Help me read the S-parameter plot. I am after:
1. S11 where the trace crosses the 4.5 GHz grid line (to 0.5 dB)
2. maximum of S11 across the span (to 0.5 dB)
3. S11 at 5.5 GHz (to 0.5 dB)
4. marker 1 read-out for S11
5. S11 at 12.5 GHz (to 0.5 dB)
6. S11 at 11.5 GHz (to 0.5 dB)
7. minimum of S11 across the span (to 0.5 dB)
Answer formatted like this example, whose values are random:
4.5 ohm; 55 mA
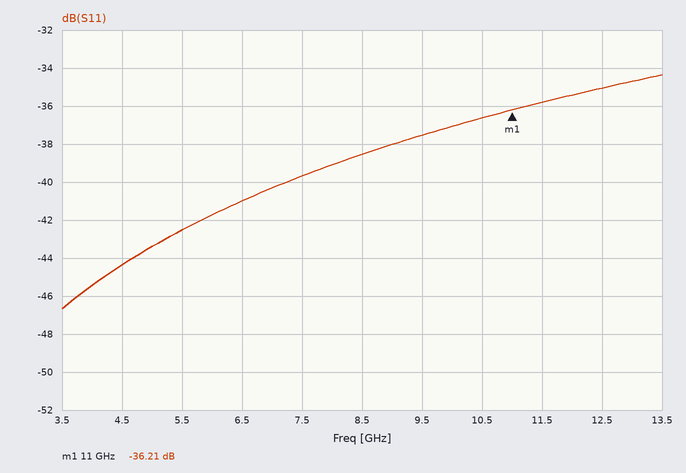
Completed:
-44.5 dB; -34.5 dB; -42.5 dB; -36.21 dB; -35.0 dB; -36.0 dB; -46.5 dB
